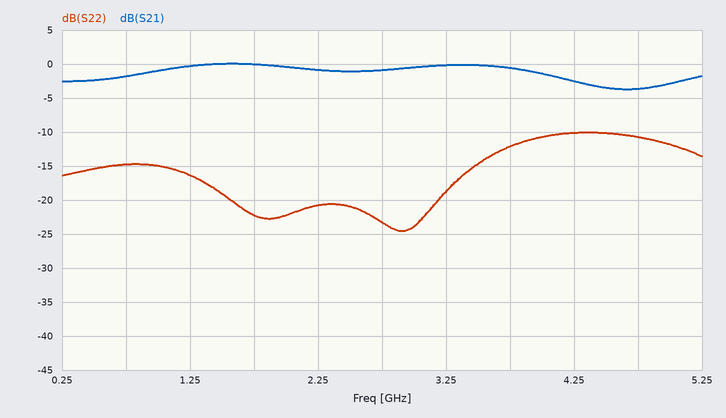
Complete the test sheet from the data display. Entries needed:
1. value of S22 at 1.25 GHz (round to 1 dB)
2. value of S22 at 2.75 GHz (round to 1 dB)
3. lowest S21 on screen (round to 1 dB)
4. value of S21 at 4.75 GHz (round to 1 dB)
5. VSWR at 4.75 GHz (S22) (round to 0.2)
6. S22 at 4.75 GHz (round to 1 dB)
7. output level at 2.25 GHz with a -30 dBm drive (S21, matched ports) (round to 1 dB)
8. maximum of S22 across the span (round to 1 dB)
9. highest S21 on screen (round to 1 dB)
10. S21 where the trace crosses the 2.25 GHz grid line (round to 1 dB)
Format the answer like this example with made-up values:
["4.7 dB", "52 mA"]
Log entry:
["-16 dB", "-23 dB", "-4 dB", "-4 dB", "1.8", "-11 dB", "-31 dBm", "-10 dB", "0 dB", "-1 dB"]
